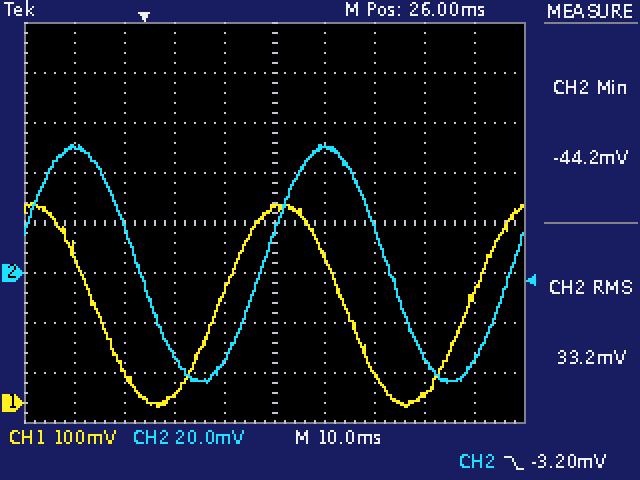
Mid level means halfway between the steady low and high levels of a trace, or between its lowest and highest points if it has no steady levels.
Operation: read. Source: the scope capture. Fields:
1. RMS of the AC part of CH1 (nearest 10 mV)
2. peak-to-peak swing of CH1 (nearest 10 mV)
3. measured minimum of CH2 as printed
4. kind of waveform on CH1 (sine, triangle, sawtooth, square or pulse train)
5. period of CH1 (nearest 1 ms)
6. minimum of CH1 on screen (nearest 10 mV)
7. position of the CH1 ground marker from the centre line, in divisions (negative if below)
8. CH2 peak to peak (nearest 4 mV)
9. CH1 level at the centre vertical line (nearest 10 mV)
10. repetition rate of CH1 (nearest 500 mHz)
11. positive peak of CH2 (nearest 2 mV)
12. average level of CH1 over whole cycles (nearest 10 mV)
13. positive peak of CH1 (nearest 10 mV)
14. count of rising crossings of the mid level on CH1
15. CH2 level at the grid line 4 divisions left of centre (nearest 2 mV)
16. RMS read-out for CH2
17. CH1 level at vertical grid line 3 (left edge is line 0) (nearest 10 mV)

140 mV
410 mV
-44.2 mV
sine
50 ms
-10 mV
-3.6 div
96 mV
390 mV
20.0 Hz
52 mV
200 mV
400 mV
2
50 mV
33.2 mV
20 mV
